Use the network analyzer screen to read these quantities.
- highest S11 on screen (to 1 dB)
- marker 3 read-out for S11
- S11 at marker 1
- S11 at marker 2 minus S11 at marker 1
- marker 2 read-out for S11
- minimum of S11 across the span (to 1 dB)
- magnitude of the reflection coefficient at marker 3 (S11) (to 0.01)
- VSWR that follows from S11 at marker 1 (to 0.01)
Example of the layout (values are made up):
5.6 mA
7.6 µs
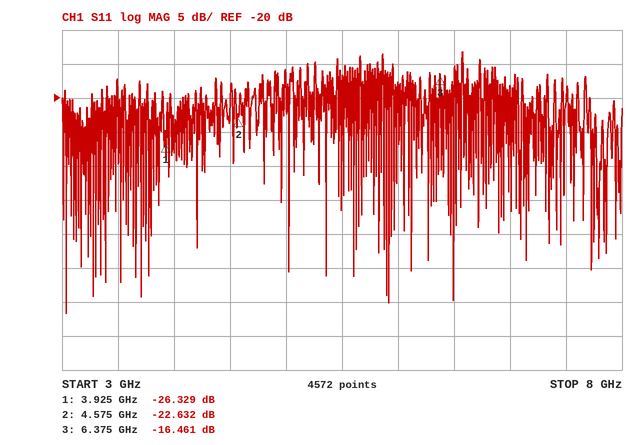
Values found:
-13 dB
-16.461 dB
-26.329 dB
3.697 dB
-22.632 dB
-52 dB
0.15
1.10
